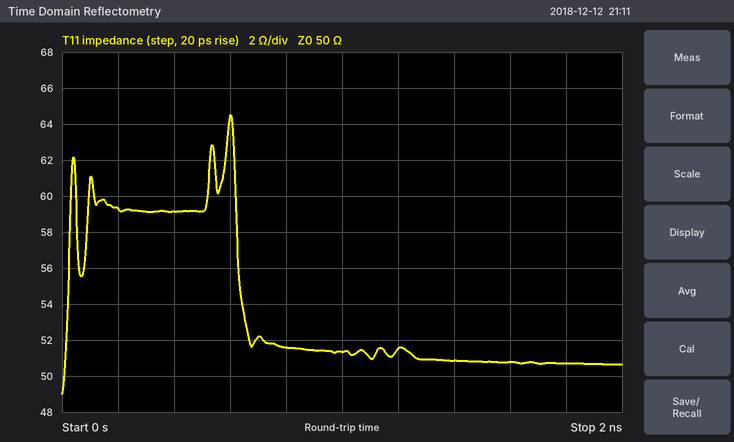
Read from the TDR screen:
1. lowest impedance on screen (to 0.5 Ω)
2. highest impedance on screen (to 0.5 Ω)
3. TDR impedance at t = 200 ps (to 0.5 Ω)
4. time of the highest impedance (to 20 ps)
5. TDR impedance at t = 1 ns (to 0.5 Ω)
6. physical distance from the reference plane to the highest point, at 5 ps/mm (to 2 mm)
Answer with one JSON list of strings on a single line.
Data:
["49.0 Ω", "64.5 Ω", "59.5 Ω", "600 ps", "51.5 Ω", "60 mm"]
